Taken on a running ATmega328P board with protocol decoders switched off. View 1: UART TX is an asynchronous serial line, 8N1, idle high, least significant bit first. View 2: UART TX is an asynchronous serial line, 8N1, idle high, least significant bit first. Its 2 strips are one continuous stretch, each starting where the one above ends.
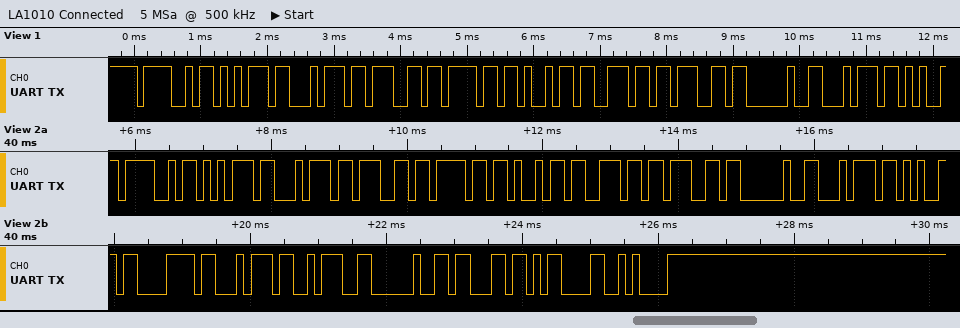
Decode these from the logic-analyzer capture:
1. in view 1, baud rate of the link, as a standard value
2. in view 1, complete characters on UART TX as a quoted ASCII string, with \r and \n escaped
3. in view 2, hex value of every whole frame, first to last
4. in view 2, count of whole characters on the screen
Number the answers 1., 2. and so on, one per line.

1. 9600 baud
2. "Outgoing t"
3. 4F 75 74 67 6F 69 6E 67 20 74 65 78 74 3A 20 63 0D 0A
4. 18
